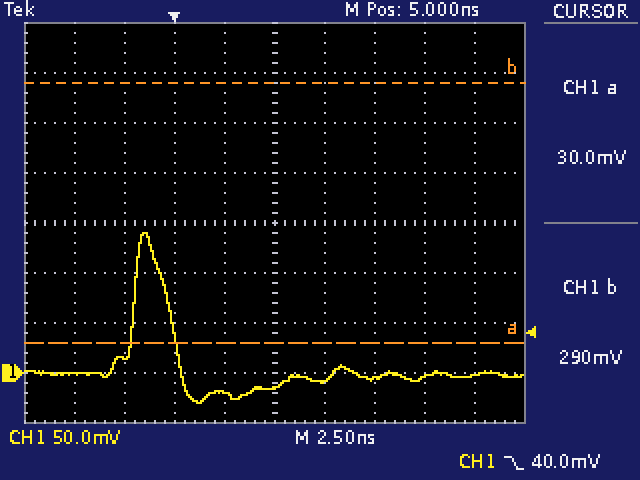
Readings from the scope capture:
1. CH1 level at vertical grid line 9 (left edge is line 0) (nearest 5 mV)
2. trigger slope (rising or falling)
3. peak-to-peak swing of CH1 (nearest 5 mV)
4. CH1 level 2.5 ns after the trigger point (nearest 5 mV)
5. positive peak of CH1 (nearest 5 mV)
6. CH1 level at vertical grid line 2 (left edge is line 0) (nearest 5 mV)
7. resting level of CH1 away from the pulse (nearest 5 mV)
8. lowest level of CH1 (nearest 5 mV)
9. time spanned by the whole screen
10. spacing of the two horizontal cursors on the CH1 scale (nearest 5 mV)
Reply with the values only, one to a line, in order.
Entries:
-5 mV
falling
170 mV
-20 mV
140 mV
15 mV
0 mV
-30 mV
25 ns
260 mV
